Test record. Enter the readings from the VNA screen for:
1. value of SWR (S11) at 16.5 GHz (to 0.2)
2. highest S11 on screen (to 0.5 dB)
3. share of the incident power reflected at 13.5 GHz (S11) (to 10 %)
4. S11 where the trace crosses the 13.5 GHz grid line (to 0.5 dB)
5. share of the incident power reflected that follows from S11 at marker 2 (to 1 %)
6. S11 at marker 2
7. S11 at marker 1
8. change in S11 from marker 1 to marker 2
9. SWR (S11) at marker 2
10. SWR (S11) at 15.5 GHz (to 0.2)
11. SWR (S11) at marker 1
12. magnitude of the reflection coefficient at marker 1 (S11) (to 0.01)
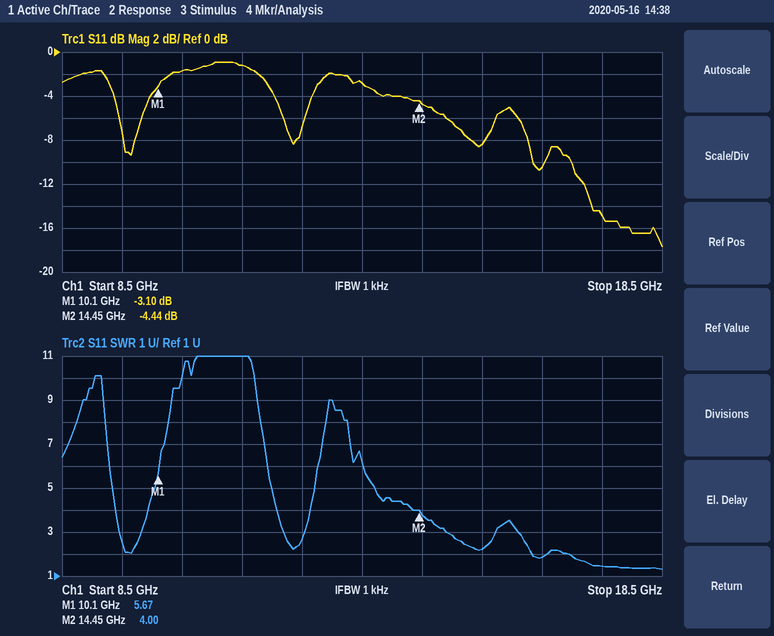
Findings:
1.8
-1.0 dB
50 %
-3.0 dB
36 %
-4.44 dB
-3.10 dB
-1.34 dB
4.00
2.2
5.67
0.70
